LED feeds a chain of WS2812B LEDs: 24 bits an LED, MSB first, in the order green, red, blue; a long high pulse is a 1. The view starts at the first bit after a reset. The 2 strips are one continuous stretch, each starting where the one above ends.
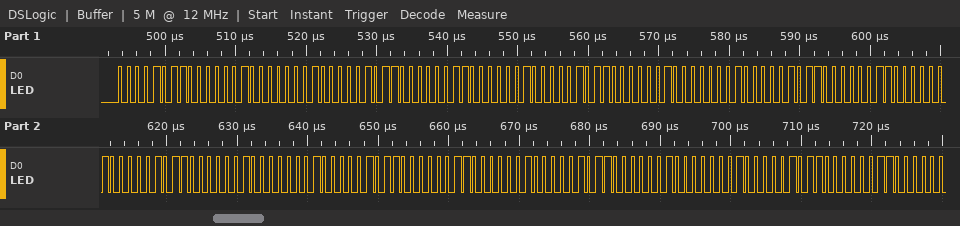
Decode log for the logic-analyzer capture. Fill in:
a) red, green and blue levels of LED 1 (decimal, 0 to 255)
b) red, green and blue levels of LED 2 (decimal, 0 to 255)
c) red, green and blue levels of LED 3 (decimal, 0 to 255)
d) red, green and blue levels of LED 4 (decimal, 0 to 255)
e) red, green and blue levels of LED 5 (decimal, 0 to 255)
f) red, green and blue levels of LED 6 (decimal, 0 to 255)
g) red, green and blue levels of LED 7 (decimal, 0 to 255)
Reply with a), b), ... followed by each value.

a) 2, 11, 2
b) 3, 11, 2
c) 2, 11, 2
d) 3, 11, 2
e) 2, 11, 2
f) 3, 11, 2
g) 2, 11, 2
